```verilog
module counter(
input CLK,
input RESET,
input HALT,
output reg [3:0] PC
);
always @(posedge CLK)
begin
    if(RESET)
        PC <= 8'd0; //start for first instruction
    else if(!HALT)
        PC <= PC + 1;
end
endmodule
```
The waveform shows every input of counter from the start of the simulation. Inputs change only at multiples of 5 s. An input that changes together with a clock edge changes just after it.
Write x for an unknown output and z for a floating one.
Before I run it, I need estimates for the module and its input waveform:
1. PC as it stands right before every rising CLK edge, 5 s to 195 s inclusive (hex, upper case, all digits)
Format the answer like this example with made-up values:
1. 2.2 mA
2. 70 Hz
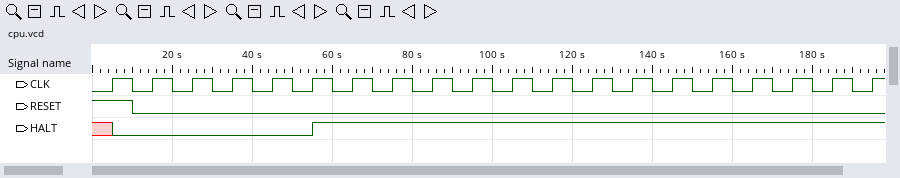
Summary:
1. x, 0, 1, 2, 3, 4, 5, 5, 5, 5, 5, 5, 5, 5, 5, 5, 5, 5, 5, 5
